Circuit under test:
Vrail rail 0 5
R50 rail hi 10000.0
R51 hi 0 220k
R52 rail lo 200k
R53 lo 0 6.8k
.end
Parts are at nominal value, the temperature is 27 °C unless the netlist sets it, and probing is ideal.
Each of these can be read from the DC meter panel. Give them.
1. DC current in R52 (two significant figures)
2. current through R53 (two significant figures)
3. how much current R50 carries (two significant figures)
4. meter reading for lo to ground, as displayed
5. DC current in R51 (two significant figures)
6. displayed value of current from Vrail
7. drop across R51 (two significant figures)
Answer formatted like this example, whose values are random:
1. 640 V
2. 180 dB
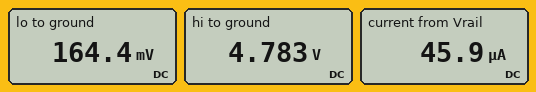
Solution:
1. 24 µA
2. 24 µA
3. 22 µA
4. 164.4 mV
5. 22 µA
6. 45.9 µA
7. 4.8 V
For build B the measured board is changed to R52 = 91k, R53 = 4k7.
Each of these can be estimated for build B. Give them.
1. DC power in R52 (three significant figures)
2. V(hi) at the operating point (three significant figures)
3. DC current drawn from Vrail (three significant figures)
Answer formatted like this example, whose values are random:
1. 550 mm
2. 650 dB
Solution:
1. 248 µW
2. 4.78 V
3. 74.0 µA
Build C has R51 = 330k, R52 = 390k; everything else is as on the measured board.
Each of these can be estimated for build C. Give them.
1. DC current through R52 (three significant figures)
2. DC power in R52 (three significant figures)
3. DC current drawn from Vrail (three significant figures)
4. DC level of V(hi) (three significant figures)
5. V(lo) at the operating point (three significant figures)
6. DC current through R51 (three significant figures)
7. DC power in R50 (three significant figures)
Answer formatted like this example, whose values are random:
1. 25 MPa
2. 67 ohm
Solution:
1. 12.6 µA
2. 61.9 µW
3. 27.3 µA
4. 4.85 V
5. 85.7 mV
6. 14.7 µA
7. 2.16 µW
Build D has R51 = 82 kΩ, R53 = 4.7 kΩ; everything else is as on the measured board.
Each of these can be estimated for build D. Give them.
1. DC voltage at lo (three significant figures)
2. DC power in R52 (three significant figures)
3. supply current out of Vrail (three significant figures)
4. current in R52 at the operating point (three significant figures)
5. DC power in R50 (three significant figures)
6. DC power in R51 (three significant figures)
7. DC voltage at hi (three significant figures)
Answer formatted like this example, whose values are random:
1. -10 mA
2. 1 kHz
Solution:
1. 115 mV
2. 119 µW
3. 78.8 µA
4. 24.4 µA
5. 29.5 µW
6. 242 µW
7. 4.46 V
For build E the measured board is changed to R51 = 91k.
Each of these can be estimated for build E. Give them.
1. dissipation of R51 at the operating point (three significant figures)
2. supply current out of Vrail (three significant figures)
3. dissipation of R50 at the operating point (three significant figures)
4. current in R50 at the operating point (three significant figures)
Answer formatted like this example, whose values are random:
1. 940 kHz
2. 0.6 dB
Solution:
1. 223 µW
2. 73.7 µA
3. 24.5 µW
4. 49.5 µA
